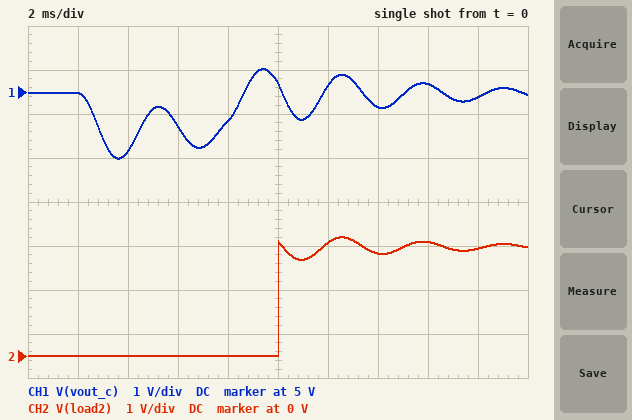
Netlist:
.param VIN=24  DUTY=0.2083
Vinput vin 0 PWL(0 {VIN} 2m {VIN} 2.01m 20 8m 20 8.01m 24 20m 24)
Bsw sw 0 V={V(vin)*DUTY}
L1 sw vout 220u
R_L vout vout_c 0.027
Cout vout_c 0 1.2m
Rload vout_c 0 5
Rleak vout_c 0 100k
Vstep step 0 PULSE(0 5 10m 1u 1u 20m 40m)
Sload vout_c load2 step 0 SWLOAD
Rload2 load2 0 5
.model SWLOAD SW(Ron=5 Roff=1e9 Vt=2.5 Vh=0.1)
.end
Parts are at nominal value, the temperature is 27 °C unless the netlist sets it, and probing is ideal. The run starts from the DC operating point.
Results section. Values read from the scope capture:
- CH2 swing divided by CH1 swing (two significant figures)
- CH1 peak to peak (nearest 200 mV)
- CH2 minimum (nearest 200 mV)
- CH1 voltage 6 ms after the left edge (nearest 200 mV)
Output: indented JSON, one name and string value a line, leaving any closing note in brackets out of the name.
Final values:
{
  "CH2 swing divided by CH1 swing": "1.3",
  "CH1 peak to peak": "2.0 V",
  "CH2 minimum": "0 V",
  "CH1 voltage 6 ms after the left edge": "4.2 V"
}
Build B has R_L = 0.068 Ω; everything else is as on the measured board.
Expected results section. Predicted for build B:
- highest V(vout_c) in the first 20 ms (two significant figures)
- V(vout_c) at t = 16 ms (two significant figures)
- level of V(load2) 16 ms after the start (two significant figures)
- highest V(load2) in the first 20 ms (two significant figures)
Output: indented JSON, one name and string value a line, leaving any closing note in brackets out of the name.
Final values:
{
  "highest V(vout_c) in the first 20 ms": "5.4 V",
  "V(vout_c) at t = 16 ms": "5.0 V",
  "level of V(load2) 16 ms after the start": "2.5 V",
  "highest V(load2) in the first 20 ms": "2.6 V"
}
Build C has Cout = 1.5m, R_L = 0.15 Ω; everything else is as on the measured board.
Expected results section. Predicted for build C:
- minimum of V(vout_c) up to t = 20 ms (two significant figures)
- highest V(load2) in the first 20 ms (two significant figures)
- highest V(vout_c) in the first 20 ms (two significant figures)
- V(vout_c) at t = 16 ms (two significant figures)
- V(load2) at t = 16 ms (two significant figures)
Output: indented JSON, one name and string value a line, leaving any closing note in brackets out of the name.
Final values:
{
  "minimum of V(vout_c) up to t = 20 ms": "3.7 V",
  "highest V(load2) in the first 20 ms": "2.6 V",
  "highest V(vout_c) in the first 20 ms": "5.3 V",
  "V(vout_c) at t = 16 ms": "4.8 V",
  "V(load2) at t = 16 ms": "2.4 V"
}
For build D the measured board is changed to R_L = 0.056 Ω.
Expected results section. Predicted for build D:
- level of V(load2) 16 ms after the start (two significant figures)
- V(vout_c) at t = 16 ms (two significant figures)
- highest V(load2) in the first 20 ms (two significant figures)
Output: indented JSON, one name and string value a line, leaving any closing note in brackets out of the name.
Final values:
{
  "level of V(load2) 16 ms after the start": "2.5 V",
  "V(vout_c) at t = 16 ms": "5.1 V",
  "highest V(load2) in the first 20 ms": "2.6 V"
}
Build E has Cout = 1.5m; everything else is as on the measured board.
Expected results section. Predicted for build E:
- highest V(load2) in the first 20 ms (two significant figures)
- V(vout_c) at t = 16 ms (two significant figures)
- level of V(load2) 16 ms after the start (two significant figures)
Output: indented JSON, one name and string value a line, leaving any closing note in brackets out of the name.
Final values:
{
  "highest V(load2) in the first 20 ms": "2.8 V",
  "V(vout_c) at t = 16 ms": "5.0 V",
  "level of V(load2) 16 ms after the start": "2.5 V"
}
